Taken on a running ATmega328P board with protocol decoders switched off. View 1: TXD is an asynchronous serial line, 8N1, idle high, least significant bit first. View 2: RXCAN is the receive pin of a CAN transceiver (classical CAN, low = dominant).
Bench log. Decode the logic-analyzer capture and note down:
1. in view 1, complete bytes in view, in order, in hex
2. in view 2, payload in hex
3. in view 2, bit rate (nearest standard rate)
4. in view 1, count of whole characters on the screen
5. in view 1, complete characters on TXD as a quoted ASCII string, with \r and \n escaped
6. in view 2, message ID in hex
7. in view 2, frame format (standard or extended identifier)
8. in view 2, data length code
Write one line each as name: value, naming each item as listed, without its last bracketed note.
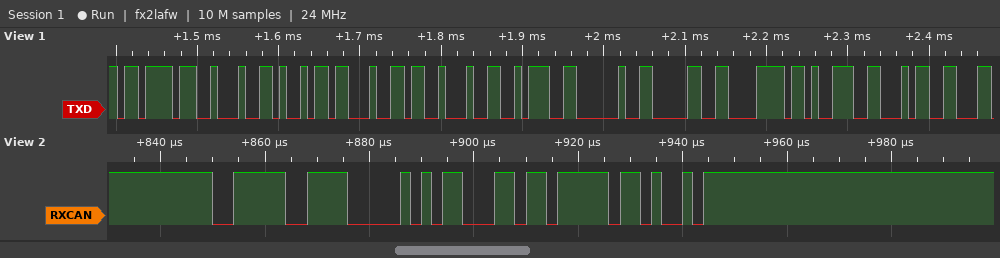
in view 1, complete bytes in view, in order, in hex: 0x7B 0x22 0x69 0x64 0x22 0x3A 0x20 0x30 0x78 0x39 0x34
in view 2, payload in hex: 63
in view 2, bit rate: 500 kbit/s
in view 1, count of whole characters on the screen: 11
in view 1, complete characters on TXD as a quoted ASCII string, with \r and \n escaped: "{\"id\": 0x94"
in view 2, message ID in hex: 0x3EF
in view 2, frame format: standard
in view 2, data length code: 1
